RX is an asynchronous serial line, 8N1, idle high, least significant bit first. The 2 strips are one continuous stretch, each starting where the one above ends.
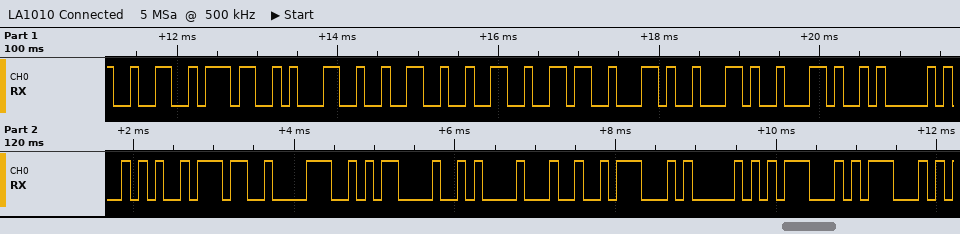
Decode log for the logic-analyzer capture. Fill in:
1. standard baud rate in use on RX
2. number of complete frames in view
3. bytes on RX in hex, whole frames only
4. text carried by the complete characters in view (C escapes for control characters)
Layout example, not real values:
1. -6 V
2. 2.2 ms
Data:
1. 9600 baud
2. 20
3. 32 37 31 32 32 36 2C 2C 2C 41 2A 37 38 0D 0A 24 47 50 47 47
4. "271226,,,A*78\r\n$GPGG"
